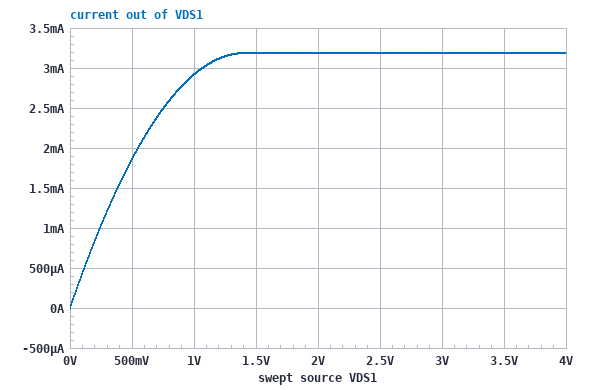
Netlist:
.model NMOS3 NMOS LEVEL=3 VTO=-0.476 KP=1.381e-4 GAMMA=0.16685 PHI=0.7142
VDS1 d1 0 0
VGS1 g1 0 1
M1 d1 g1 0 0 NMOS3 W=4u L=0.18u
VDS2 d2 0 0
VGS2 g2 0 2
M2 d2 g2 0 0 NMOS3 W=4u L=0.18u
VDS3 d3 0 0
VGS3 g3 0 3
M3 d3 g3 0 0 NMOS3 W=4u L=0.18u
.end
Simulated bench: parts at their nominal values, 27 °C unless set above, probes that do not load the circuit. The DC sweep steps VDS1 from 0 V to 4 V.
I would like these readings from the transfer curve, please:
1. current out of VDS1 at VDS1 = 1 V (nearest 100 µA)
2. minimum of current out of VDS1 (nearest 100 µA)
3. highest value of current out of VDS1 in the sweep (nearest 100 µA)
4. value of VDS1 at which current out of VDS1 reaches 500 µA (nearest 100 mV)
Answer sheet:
2.9 mA
0 A
3.2 mA
100 mV
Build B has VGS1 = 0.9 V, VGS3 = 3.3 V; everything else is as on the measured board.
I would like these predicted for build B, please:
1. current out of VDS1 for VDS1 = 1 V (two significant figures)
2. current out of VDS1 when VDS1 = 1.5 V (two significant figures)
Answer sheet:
2.6 mA
2.8 mA
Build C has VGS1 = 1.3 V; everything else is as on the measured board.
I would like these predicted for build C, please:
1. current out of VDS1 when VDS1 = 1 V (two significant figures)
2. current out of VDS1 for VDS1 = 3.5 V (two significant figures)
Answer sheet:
3.8 mA
4.6 mA
